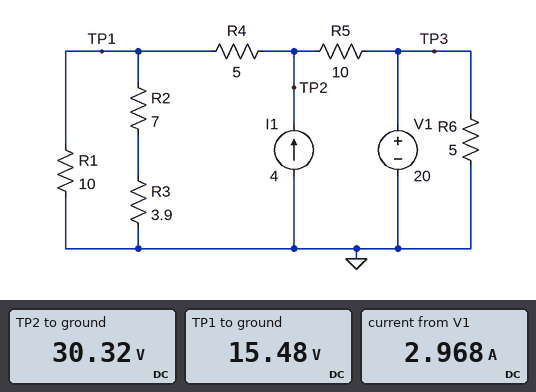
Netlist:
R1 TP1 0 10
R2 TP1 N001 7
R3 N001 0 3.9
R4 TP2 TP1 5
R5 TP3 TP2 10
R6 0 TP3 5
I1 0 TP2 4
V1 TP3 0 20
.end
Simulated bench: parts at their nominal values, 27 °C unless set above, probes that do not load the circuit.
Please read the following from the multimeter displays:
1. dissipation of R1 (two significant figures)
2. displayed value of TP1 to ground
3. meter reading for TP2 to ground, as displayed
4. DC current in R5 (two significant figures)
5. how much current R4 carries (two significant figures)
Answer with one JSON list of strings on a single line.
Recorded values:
["24 W", "15.48 V", "30.32 V", "1.0 A", "3.0 A"]
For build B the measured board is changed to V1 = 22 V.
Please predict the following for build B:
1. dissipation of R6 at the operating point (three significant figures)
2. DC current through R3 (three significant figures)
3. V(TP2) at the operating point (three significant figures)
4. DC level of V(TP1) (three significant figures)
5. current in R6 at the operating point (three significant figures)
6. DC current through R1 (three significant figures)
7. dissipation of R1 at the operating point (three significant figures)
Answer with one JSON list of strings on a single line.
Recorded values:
["96.8 W", "1.47 A", "31.3 V", "16.0 V", "4.40 A", "1.60 A", "25.6 W"]
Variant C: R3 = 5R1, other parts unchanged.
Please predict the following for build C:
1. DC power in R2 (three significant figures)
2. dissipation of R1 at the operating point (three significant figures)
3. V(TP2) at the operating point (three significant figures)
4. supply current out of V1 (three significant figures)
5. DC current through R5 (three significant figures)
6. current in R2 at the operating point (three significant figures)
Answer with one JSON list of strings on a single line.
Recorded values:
["12.3 W", "25.7 W", "30.7 V", "2.93 A", "1.07 A", "1.33 A"]
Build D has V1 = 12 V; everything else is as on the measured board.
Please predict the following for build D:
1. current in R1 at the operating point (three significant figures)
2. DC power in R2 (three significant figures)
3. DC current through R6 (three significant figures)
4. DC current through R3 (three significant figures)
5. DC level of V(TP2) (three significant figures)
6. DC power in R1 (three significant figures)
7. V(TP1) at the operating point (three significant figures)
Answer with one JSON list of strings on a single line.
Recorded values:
["1.34 A", "10.6 W", "2.40 A", "1.23 A", "26.3 V", "18.0 W", "13.4 V"]
